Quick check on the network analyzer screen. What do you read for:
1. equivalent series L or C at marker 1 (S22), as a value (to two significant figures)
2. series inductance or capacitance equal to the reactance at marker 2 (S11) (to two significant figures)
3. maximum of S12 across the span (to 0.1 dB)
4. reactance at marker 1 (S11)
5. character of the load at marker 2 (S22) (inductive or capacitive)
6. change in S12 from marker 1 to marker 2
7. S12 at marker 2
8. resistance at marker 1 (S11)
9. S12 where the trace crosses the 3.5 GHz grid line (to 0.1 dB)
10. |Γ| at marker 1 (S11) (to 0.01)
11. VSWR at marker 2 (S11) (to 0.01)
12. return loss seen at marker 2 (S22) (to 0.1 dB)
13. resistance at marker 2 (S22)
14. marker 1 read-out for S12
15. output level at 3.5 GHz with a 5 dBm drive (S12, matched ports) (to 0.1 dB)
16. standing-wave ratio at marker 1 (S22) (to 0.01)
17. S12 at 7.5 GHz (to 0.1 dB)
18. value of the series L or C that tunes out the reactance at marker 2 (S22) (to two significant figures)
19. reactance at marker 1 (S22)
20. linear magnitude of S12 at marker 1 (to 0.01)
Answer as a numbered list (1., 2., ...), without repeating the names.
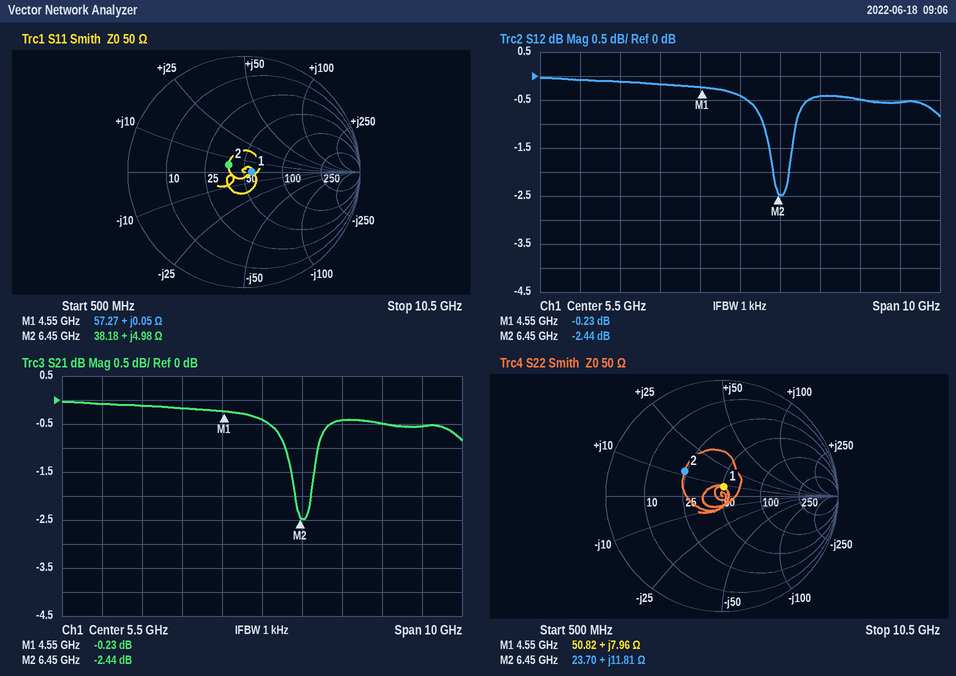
1. 280 pH
2. 120 pH
3. 0.0 dB
4. +0.05 Ω
5. inductive
6. -2.21 dB
7. -2.44 dB
8. 57.27 Ω
9. -0.2 dB
10. 0.07
11. 1.34
12. 8.3 dB
13. 23.70 Ω
14. -0.23 dB
15. 4.8 dBm
16. 1.17
17. -0.4 dB
18. 2.1 pF
19. +7.96 Ω
20. 0.97
